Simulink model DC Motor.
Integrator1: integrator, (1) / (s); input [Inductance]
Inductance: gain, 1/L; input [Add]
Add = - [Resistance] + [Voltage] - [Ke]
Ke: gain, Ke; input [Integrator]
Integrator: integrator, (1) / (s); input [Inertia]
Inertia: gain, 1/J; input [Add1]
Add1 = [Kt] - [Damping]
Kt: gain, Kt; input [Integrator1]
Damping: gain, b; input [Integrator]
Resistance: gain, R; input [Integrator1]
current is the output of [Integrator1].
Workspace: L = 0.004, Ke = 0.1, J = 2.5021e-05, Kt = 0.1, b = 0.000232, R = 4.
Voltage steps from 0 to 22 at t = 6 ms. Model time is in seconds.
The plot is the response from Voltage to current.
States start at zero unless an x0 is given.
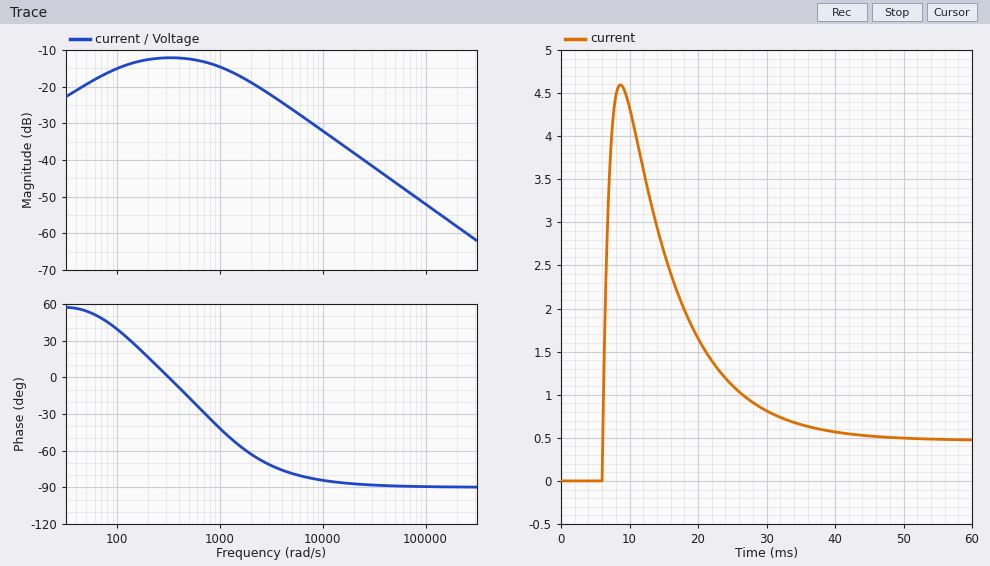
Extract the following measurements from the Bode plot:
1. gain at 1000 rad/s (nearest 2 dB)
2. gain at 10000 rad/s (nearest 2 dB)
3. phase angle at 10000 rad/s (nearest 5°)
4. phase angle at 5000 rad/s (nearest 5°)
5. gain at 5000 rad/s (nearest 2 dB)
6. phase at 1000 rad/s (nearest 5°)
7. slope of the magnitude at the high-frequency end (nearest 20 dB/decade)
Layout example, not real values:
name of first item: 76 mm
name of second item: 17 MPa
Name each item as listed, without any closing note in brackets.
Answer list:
gain at 1000 rad/s: -14 dB
gain at 10000 rad/s: -32 dB
phase angle at 10000 rad/s: -85°
phase angle at 5000 rad/s: -80°
gain at 5000 rad/s: -26 dB
phase at 1000 rad/s: -40°
slope of the magnitude at the high-frequency end: -20 dB/decade
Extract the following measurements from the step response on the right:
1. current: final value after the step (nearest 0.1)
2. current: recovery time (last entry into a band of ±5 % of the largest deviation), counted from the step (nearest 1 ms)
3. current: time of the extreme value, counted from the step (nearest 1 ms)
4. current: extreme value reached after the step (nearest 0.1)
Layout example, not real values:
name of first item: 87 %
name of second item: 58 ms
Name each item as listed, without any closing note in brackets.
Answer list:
current: final value after the step: 0.5
current: recovery time (last entry into a band of ±5 % of the largest deviation), counted from the step: 27 ms
current: time of the extreme value, counted from the step: 3 ms
current: extreme value reached after the step: 4.6
